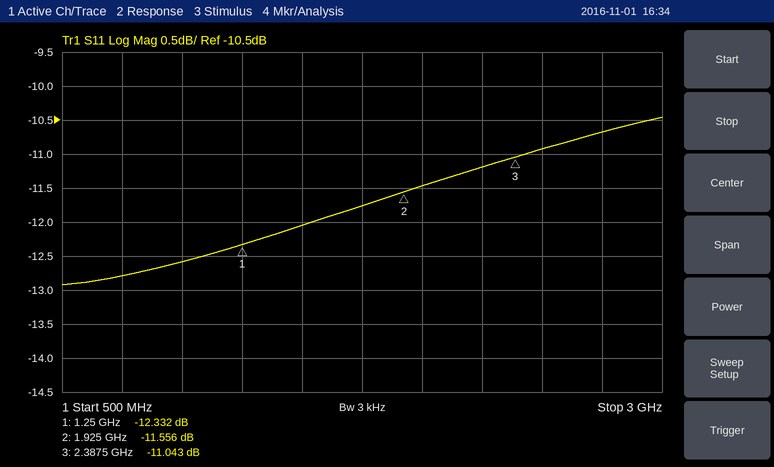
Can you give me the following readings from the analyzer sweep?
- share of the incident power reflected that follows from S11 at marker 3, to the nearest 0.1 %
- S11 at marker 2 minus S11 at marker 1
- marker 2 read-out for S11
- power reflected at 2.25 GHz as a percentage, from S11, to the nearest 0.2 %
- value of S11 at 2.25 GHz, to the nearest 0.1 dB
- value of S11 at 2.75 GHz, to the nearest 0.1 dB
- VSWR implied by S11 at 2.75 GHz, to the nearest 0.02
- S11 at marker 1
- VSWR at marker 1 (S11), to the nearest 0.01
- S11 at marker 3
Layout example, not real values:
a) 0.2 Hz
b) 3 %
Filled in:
a) 7.9 %
b) 0.776 dB
c) -11.556 dB
d) 7.6 %
e) -11.2 dB
f) -10.7 dB
g) 1.82
h) -12.332 dB
i) 1.64
j) -11.043 dB
